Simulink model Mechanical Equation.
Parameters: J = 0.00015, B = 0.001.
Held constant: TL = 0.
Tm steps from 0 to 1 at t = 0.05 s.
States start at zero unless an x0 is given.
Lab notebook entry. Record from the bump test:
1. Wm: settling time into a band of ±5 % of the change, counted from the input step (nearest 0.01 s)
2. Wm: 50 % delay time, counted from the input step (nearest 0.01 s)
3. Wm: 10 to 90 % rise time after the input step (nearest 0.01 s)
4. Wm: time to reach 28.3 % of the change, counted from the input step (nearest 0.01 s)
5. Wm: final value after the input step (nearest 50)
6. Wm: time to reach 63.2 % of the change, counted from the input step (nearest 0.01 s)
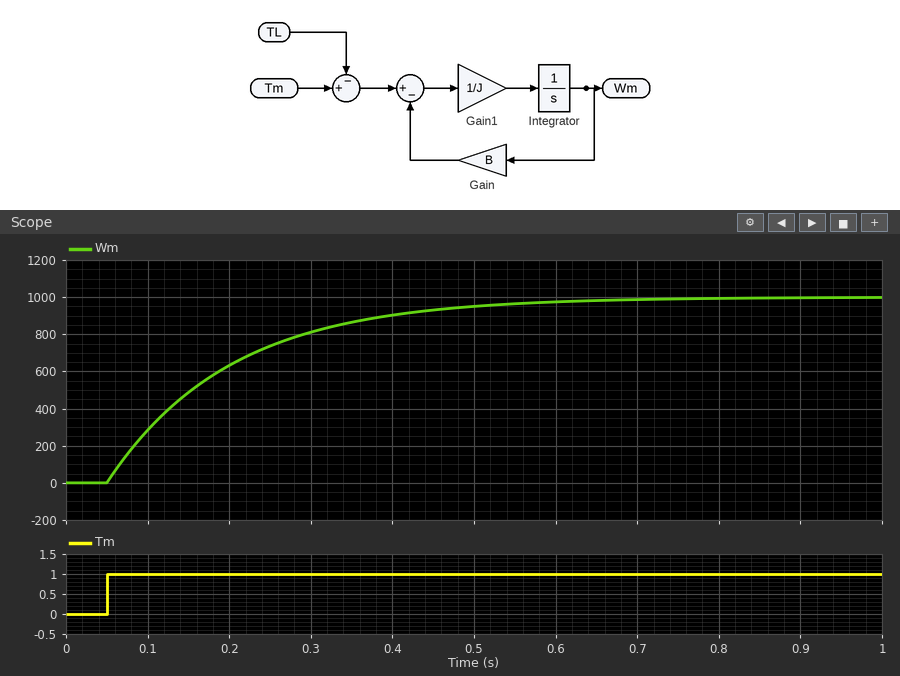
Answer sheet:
0.45 s
0.10 s
0.33 s
0.05 s
1000
0.15 s
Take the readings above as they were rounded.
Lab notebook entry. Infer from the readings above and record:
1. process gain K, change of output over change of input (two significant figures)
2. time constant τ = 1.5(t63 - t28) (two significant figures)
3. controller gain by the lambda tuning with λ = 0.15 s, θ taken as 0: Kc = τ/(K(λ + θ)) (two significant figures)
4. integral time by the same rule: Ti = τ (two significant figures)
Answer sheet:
1000
0.15 s
0.0010
0.15 s
